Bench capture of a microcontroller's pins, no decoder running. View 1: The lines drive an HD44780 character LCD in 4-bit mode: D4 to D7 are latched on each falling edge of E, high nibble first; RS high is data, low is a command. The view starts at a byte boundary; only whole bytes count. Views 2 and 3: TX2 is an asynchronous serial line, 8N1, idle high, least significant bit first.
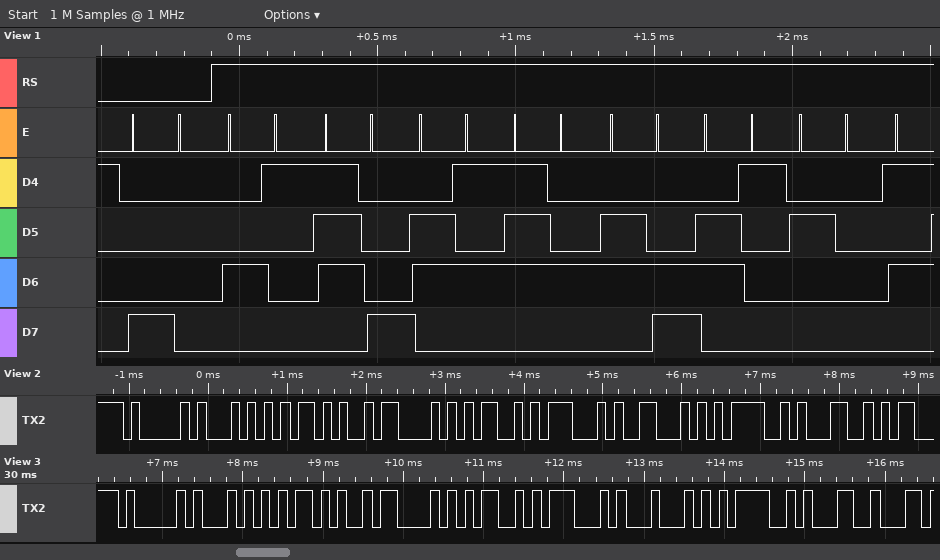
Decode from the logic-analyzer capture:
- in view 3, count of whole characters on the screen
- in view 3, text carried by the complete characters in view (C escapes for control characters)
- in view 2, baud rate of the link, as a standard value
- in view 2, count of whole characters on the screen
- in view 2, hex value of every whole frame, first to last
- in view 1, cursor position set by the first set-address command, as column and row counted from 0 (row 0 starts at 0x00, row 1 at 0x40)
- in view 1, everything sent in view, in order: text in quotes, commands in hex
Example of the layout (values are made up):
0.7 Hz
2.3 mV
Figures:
9
"AT+CMGD=1"
9600 baud
9
0x41 0x54 0x2B 0x43 0x4D 0x47 0x46 0x3D 0x31
column 0, row 0
0x80 "Axetla "
